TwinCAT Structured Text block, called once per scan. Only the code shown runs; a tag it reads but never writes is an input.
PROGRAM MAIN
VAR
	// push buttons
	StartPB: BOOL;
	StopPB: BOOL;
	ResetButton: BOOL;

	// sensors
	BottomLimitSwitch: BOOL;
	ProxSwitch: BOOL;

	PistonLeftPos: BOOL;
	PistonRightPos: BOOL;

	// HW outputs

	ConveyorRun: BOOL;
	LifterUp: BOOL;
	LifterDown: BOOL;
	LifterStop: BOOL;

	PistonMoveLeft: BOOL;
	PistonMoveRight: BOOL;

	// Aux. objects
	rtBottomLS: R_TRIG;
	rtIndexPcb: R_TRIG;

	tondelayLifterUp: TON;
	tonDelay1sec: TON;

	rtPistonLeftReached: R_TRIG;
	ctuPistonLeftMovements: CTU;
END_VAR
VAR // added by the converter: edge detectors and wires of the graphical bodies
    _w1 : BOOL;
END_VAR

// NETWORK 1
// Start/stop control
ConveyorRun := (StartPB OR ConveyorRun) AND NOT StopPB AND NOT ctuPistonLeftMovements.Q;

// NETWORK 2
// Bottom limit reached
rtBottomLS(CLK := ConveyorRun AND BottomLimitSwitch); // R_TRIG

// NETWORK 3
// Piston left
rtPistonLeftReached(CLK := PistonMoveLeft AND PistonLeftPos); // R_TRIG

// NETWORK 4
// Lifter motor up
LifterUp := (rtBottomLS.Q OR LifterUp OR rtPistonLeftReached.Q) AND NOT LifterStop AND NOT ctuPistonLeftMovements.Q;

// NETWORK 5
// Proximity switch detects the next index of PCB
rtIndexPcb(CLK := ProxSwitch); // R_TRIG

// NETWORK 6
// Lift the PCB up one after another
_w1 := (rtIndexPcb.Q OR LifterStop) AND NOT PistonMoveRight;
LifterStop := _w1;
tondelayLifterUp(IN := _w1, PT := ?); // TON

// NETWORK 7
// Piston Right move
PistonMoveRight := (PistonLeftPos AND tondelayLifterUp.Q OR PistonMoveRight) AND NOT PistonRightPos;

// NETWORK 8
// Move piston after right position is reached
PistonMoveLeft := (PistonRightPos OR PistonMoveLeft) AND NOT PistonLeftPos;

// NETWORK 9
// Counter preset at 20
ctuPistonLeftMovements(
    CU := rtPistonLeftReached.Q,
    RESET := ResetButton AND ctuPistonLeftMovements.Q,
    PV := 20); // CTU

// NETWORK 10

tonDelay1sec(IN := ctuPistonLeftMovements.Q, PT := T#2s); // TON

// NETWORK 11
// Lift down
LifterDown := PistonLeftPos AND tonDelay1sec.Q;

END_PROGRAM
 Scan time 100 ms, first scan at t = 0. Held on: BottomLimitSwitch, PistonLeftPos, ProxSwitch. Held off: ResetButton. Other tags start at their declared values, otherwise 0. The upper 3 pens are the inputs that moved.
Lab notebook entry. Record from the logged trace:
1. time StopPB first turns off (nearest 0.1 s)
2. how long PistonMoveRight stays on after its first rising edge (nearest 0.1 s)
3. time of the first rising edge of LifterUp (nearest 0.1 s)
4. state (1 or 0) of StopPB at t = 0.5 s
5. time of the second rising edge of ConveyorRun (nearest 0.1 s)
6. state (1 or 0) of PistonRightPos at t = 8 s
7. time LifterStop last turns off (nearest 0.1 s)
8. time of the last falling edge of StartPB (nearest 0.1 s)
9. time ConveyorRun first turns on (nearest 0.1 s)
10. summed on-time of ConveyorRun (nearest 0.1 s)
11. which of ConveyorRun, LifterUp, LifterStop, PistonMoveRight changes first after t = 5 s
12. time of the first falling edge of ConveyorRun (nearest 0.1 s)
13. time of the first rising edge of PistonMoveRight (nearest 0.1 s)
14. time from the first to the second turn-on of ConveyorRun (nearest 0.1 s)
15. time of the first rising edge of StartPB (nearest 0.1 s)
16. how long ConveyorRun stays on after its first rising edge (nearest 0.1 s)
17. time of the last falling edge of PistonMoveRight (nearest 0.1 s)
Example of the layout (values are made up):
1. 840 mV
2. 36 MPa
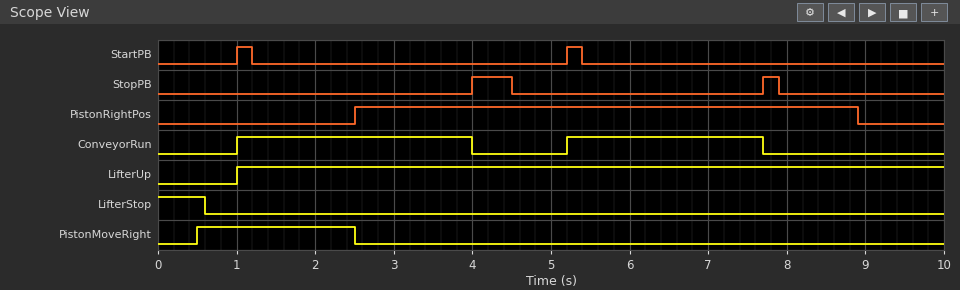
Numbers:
1. 4.5 s
2. 2.0 s
3. 1.0 s
4. 0
5. 5.2 s
6. 1
7. 0.6 s
8. 5.4 s
9. 1.0 s
10. 5.5 s
11. ConveyorRun
12. 4.0 s
13. 0.5 s
14. 4.2 s
15. 1.0 s
16. 3.0 s
17. 2.5 s
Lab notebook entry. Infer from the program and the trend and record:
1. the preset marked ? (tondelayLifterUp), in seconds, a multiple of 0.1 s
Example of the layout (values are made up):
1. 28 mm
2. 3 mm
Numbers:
1. 0.5 s
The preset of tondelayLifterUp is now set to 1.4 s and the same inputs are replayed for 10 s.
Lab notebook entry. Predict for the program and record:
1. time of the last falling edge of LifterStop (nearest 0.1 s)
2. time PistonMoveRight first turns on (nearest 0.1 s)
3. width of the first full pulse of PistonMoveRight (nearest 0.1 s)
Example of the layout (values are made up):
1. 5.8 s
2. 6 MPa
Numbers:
1. 1.5 s
2. 1.4 s
3. 1.1 s
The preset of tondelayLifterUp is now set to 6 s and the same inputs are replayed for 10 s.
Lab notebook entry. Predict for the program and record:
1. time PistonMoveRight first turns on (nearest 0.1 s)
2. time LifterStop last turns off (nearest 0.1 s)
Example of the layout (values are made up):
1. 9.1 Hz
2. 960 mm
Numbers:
1. 8.9 s
2. 9.0 s
